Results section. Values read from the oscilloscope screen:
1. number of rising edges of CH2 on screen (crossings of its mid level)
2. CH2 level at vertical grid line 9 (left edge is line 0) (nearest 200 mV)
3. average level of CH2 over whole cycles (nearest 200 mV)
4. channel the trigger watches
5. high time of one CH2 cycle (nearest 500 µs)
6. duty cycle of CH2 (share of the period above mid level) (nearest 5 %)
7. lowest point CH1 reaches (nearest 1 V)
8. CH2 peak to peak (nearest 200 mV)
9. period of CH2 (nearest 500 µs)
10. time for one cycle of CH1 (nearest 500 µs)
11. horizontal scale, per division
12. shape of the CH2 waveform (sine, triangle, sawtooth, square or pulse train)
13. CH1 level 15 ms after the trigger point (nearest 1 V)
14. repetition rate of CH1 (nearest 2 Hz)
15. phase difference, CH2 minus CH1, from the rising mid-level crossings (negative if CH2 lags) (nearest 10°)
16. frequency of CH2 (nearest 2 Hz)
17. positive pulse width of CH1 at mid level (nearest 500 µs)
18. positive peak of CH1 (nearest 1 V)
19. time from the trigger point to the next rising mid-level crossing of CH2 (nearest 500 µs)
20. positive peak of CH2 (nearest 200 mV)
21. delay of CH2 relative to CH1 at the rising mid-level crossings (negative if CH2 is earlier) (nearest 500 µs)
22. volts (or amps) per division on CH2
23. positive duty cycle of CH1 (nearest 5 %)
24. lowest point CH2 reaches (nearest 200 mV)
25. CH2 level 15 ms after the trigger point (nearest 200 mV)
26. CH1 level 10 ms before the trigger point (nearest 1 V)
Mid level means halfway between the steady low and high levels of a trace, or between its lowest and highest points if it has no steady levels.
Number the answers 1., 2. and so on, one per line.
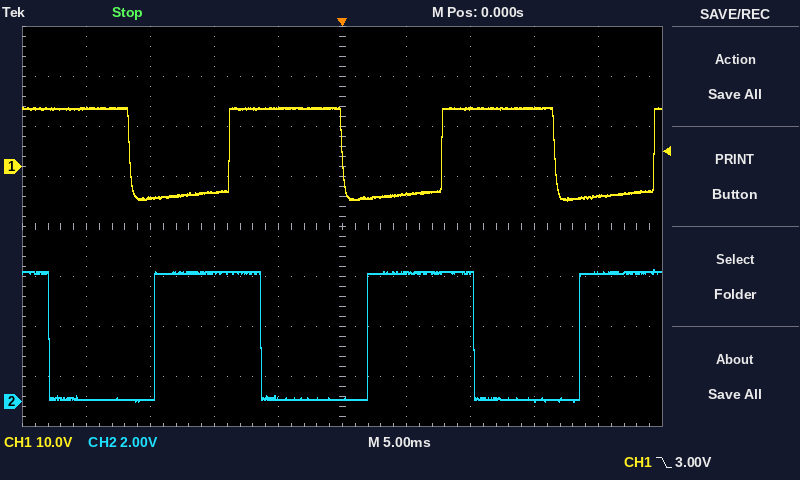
1. 3
2. 5.2 V
3. 2.6 V
4. CH1
5. 8.5 ms
6. 50 %
7. -7 V
8. 5.2 V
9. 16.5 ms
10. 16.5 ms
11. 5 ms
12. square
13. 12 V
14. 60 Hz
15. +130°
16. 60 Hz
17. 9.0 ms
18. 12 V
19. 2.0 ms
20. 5.2 V
21. -6.0 ms
22. 2 V
23. 55 %
24. 0.0 V
25. 0.0 V
26. -5 V
